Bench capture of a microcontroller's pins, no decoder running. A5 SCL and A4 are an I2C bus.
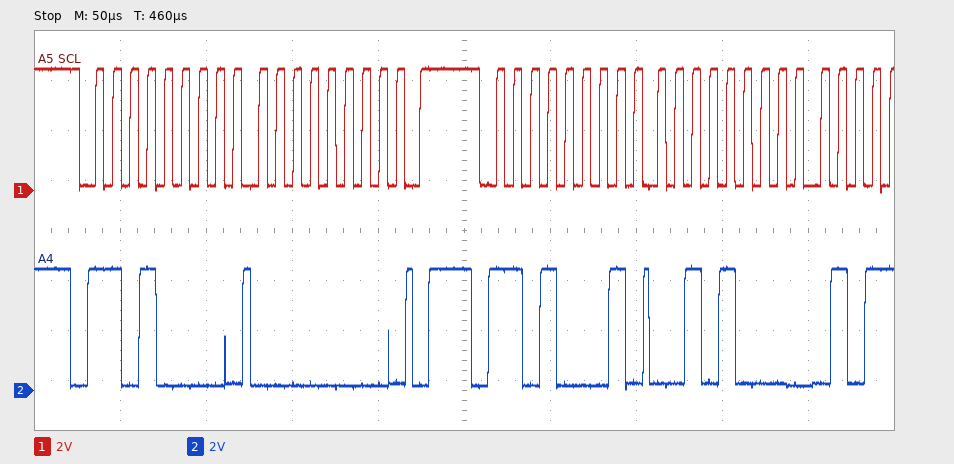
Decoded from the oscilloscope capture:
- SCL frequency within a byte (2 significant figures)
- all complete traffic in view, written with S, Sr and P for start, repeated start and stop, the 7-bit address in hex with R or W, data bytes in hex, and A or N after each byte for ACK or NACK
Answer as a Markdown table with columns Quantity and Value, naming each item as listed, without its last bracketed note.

| Quantity | Value |
|---|---|
| SCL frequency within a byte | 100 kHz |
| all complete traffic in view, written with S, Sr and P for start, repeated start and stop, the 7-bit address in hex with R or W, data bytes in hex, and A or N after each byte for ACK or NACK | S 68W A 00 A P S 68R A 28 A |
